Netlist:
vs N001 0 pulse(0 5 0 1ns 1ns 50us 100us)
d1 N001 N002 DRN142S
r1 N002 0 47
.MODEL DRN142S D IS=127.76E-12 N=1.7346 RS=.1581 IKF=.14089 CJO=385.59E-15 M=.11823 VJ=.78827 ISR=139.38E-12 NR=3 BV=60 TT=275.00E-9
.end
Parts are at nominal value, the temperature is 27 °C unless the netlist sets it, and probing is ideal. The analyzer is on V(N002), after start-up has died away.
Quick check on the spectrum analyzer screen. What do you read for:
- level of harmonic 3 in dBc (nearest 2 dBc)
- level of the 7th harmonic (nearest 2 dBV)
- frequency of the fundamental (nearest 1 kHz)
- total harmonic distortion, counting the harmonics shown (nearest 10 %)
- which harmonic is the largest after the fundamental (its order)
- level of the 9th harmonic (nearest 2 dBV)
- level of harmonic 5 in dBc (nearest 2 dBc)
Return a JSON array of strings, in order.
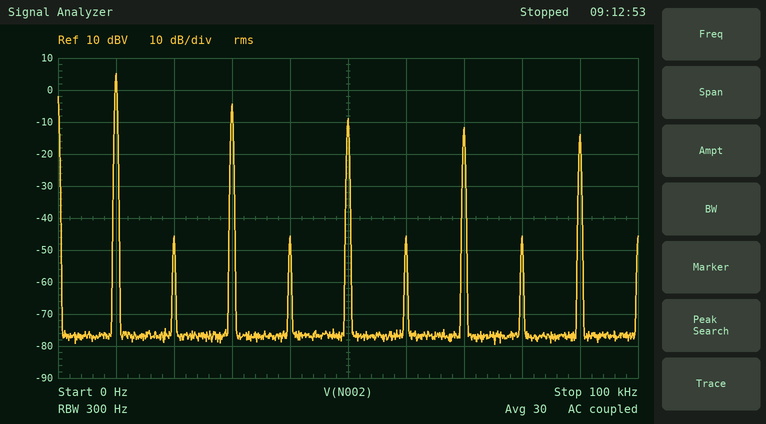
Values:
["-10 dBc", "-12 dBV", "10 kHz", "40 %", "3", "-14 dBV", "-14 dBc"]
